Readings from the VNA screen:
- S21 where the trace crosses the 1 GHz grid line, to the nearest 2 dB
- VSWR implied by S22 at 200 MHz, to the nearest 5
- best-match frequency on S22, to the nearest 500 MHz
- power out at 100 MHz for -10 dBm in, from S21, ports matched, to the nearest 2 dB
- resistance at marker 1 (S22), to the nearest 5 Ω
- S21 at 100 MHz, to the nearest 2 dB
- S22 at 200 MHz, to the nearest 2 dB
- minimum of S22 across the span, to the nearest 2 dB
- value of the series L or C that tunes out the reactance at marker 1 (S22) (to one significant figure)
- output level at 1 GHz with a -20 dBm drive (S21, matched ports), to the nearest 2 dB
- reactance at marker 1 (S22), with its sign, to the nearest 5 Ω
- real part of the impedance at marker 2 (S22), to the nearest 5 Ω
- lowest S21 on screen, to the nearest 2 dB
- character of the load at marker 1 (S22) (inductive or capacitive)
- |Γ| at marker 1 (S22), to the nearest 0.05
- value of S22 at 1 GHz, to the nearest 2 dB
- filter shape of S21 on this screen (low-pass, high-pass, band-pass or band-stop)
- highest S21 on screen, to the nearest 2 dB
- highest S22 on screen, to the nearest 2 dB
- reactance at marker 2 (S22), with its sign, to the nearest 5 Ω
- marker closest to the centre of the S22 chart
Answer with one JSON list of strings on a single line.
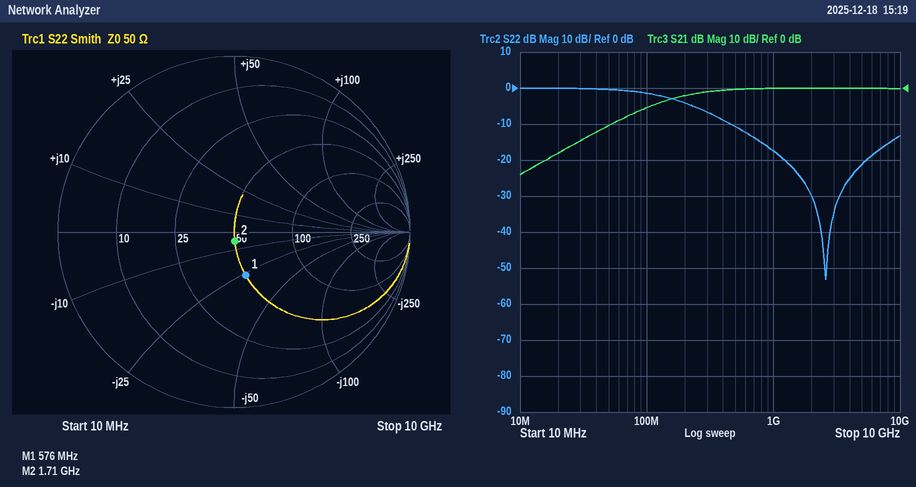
["0 dB", "5", "2.5 GHz", "-16 dBm", "50 Ω", "-6 dB", "-4 dB", "-54 dB", "7 nH", "-20 dBm", "-25 Ω", "50 Ω", "-24 dB", "capacitive", "0.25", "-18 dB", "high-pass", "0 dB", "0 dB", "-5 Ω", "marker 2"]
